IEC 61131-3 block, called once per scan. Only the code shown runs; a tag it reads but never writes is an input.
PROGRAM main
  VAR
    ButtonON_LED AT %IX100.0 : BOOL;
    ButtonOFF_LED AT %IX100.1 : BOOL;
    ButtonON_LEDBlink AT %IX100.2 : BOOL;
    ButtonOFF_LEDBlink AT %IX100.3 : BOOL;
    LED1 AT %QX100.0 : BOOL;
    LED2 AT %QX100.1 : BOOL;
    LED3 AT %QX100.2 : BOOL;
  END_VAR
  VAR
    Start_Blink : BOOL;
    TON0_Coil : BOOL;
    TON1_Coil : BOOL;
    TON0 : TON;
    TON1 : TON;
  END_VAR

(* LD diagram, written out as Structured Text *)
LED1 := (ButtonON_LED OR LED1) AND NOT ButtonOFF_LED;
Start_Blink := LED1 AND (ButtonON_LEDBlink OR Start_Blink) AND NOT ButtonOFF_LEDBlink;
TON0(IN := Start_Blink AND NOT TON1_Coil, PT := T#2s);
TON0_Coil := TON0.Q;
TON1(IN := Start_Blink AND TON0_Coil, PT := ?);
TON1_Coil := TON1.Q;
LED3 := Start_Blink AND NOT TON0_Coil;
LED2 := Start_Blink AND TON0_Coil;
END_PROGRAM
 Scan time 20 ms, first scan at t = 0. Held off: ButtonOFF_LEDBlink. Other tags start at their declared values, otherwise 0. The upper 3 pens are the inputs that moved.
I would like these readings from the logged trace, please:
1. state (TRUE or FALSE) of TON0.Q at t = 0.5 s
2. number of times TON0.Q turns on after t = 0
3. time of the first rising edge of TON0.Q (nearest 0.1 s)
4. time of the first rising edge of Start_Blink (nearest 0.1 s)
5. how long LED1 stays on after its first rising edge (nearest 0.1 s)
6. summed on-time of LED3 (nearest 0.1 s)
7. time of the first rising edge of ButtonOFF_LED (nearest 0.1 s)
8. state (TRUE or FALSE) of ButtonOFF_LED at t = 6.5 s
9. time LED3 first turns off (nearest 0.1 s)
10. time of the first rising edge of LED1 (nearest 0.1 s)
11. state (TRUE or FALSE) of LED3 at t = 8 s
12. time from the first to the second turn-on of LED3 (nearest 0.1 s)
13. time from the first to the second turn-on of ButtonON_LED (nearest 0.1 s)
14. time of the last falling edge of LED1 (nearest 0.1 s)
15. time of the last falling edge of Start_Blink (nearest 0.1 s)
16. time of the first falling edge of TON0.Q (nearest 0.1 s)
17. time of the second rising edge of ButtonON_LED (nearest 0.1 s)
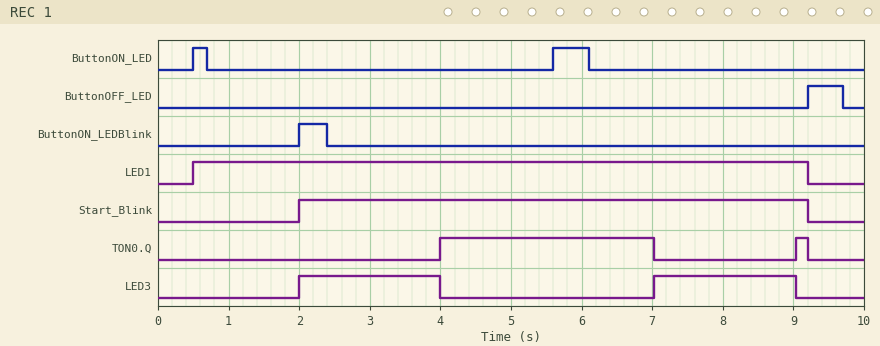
FALSE
2
4.0 s
2.0 s
8.7 s
4.0 s
9.2 s
FALSE
4.0 s
0.5 s
TRUE
5.0 s
5.1 s
9.2 s
9.2 s
7.0 s
5.6 s
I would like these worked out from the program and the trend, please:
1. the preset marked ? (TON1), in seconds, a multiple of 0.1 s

3.0 s
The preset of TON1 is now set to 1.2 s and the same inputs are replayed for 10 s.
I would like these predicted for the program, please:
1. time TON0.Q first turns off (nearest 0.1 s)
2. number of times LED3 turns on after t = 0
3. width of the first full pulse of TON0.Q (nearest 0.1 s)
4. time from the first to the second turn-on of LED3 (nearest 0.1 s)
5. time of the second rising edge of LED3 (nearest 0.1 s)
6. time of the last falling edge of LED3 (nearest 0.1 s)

5.2 s
3
1.2 s
3.2 s
5.2 s
9.2 s
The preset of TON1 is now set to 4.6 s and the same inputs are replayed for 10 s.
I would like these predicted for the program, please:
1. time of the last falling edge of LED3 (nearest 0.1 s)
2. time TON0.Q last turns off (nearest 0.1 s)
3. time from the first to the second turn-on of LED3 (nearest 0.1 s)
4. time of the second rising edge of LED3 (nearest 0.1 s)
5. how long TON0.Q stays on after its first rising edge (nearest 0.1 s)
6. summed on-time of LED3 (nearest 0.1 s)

9.2 s
8.6 s
6.6 s
8.6 s
4.6 s
2.6 s
